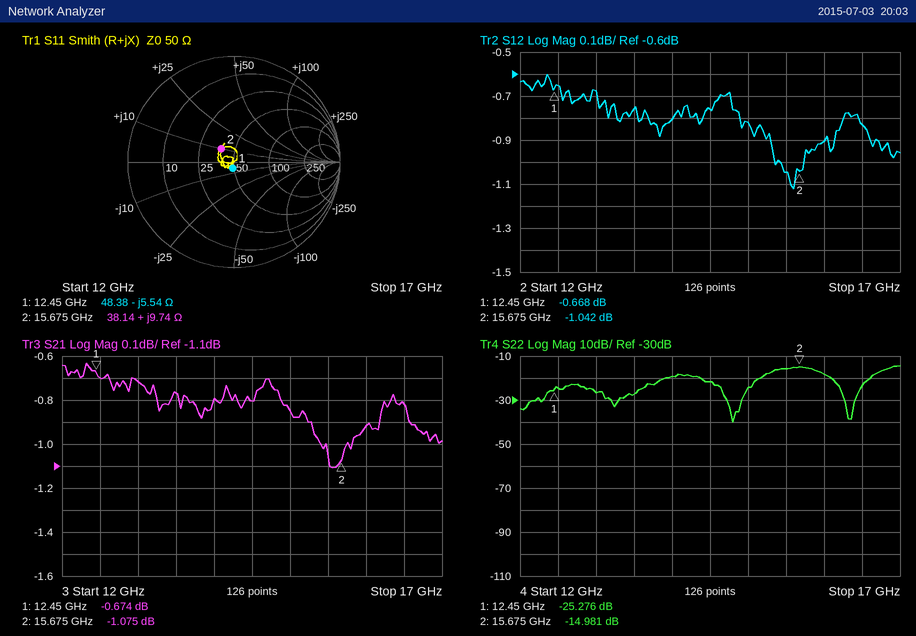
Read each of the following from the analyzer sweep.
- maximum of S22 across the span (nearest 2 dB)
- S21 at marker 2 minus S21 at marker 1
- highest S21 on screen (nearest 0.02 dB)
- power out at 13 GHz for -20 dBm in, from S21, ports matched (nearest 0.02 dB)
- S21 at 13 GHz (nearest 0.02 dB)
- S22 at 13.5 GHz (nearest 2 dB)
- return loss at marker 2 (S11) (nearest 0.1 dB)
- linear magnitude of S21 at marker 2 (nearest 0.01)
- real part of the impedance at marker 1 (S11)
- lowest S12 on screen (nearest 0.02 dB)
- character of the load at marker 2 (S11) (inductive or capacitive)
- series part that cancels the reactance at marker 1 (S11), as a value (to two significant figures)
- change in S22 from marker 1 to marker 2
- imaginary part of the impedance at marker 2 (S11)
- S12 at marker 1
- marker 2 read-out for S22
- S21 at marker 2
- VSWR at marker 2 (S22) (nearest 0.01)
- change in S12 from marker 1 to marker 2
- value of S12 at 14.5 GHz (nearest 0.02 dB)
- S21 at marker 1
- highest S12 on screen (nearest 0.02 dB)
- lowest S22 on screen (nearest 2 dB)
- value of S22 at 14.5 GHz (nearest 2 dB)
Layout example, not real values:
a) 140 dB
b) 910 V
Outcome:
a) -14 dB
b) -0.401 dB
c) -0.64 dB
d) -20.72 dBm
e) -0.72 dB
f) -28 dB
g) 15.2 dB
h) 0.88
i) 48.38 Ω
j) -1.12 dB
k) inductive
l) 71 pH
m) 10.295 dB
n) +9.74 Ω
o) -0.668 dB
p) -14.981 dB
q) -1.075 dB
r) 1.43
s) -0.374 dB
t) -0.76 dB
u) -0.674 dB
v) -0.60 dB
w) -40 dB
x) -22 dB
